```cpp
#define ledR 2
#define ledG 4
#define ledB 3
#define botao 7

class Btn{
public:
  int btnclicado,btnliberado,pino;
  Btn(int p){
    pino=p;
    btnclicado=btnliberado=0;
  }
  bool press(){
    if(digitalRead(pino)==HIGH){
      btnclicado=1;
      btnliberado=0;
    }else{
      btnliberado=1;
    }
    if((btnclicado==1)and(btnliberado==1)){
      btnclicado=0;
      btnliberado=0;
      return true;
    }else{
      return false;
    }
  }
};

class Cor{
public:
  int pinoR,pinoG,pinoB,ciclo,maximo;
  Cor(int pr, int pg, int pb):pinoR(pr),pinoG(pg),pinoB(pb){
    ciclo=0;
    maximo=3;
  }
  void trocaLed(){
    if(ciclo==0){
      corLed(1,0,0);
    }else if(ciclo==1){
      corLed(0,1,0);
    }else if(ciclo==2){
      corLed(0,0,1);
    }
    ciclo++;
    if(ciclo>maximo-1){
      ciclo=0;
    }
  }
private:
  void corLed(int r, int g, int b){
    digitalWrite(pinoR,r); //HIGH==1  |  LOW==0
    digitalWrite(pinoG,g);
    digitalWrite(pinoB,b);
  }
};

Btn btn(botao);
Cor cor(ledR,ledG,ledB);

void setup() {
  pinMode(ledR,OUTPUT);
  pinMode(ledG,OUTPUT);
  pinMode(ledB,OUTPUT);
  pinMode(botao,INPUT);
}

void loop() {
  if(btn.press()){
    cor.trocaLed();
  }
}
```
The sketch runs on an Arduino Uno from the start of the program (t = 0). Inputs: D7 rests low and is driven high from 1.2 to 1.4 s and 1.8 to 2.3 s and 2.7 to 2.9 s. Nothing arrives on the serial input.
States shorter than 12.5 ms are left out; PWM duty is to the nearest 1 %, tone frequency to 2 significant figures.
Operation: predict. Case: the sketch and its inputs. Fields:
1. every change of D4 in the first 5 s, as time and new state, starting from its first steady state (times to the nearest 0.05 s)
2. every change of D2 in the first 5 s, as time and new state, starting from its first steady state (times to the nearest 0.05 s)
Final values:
0 s low; 2.3 s high; 2.9 s low
0 s low; 1.4 s high; 2.3 s low
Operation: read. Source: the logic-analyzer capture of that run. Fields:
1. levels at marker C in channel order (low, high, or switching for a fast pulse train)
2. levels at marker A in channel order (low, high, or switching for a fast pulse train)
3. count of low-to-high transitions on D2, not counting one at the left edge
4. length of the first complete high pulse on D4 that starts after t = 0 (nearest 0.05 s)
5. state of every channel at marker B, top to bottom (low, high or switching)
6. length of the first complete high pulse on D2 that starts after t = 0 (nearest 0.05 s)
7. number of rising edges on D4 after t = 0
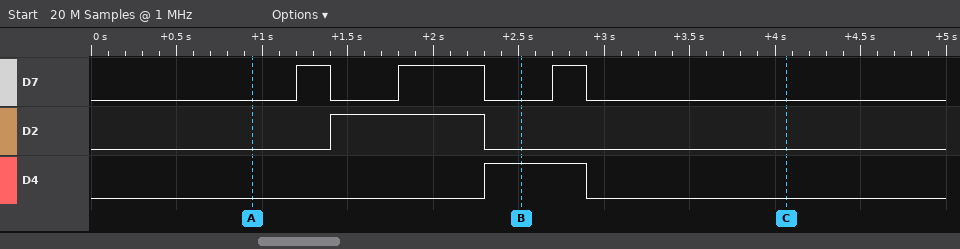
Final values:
D7 low, D2 low, D4 low
D7 low, D2 low, D4 low
1
0.60 s
D7 low, D2 low, D4 high
0.90 s
1
